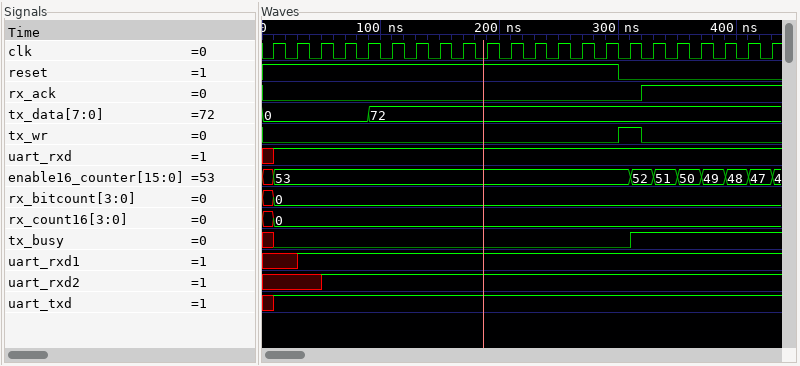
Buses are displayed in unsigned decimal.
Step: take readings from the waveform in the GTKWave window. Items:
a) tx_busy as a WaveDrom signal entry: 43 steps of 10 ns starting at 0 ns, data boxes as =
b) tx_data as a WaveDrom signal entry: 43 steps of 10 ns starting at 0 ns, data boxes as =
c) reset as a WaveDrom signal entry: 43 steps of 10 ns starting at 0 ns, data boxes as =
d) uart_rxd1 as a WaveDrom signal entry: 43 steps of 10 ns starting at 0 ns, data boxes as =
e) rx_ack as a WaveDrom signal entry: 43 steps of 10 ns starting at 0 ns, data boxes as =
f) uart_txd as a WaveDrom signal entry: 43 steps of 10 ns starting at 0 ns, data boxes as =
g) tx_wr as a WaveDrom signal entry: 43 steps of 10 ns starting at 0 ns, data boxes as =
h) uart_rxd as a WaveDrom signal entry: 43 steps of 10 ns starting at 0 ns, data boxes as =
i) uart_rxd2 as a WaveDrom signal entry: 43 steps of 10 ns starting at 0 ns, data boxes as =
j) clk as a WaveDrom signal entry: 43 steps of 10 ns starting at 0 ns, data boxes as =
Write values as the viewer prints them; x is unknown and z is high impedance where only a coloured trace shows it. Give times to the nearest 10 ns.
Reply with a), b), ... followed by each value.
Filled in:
a) {name: 'tx_busy', wave: 'x0.............................1...........'}
b) {name: 'tx_data', wave: '=........=.................................', data: '0 72'}
c) {name: 'reset', wave: '1.............................0............'}
d) {name: 'uart_rxd1', wave: 'x..1.......................................'}
e) {name: 'rx_ack', wave: '0...............................1..........'}
f) {name: 'uart_txd', wave: 'x1.........................................'}
g) {name: 'tx_wr', wave: '0.............................1.0..........'}
h) {name: 'uart_rxd', wave: 'x1.........................................'}
i) {name: 'uart_rxd2', wave: 'x....1.....................................'}
j) {name: 'clk', wave: '0101010101010101010101010101010101010101010'}
